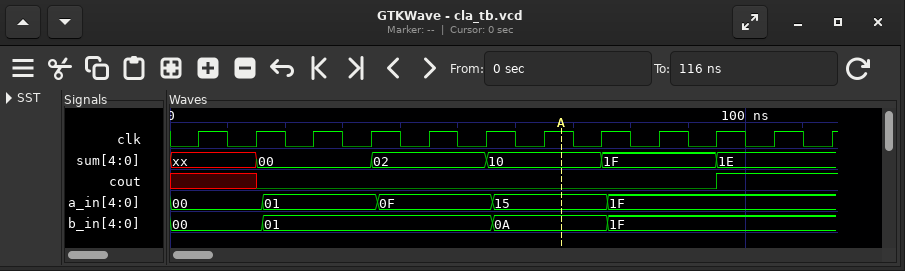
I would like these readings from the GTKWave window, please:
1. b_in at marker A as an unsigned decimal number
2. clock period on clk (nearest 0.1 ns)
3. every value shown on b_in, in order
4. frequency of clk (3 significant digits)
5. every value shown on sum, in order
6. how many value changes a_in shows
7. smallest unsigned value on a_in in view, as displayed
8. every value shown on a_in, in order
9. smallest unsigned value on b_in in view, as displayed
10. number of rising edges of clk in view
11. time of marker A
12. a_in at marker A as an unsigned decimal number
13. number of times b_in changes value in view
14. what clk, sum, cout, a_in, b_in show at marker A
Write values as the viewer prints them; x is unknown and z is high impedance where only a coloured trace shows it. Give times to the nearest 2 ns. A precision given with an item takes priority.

10
10 ns
00, 01, 0A, 1F
100 MHz
xx, 00, 02, 10, 1F, 1E
4
00
00, 01, 0F, 15, 1F
00
12
68 ns
21
3
clk=1, sum=10, cout=0, a_in=15, b_in=0A
